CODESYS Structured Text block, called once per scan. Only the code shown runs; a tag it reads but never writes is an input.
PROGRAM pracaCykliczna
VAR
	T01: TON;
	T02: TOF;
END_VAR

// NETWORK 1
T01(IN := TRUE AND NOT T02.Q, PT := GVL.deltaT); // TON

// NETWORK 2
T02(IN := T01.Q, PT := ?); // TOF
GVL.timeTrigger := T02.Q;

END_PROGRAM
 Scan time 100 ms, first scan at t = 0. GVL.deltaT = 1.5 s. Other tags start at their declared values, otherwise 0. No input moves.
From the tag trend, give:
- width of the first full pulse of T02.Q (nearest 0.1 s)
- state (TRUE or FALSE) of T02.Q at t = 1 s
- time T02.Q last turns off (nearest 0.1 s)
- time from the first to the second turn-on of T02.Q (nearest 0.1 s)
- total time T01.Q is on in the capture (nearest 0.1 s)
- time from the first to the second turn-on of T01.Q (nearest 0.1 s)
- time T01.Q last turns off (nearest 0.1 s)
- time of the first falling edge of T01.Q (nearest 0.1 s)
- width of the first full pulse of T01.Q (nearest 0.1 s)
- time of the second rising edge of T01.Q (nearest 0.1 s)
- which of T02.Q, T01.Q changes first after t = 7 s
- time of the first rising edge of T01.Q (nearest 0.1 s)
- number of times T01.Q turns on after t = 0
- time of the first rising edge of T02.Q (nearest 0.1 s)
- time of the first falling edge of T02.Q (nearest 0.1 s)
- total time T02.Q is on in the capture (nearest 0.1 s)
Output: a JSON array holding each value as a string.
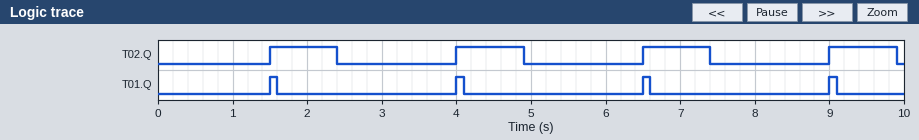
["0.9 s", "FALSE", "9.9 s", "2.5 s", "0.4 s", "2.5 s", "9.1 s", "1.6 s", "0.1 s", "4.0 s", "T02.Q", "1.5 s", "4", "1.5 s", "2.4 s", "3.6 s"]
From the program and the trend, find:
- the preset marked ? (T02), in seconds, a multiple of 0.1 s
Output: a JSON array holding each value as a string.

["0.8 s"]
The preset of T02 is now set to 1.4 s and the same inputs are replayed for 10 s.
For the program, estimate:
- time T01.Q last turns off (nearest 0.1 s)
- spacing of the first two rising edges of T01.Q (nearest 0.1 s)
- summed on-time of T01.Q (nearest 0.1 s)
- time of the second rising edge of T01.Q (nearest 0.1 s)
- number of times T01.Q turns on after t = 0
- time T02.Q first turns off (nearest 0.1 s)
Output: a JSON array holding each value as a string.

["7.8 s", "3.1 s", "0.3 s", "4.6 s", "3", "3.0 s"]
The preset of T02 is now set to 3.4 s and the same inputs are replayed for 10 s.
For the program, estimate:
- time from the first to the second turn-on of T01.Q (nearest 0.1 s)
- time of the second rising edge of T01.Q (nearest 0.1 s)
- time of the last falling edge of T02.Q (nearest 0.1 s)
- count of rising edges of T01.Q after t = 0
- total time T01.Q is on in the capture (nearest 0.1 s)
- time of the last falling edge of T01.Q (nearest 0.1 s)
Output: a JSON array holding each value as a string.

["5.1 s", "6.6 s", "5.0 s", "2", "0.2 s", "6.7 s"]
